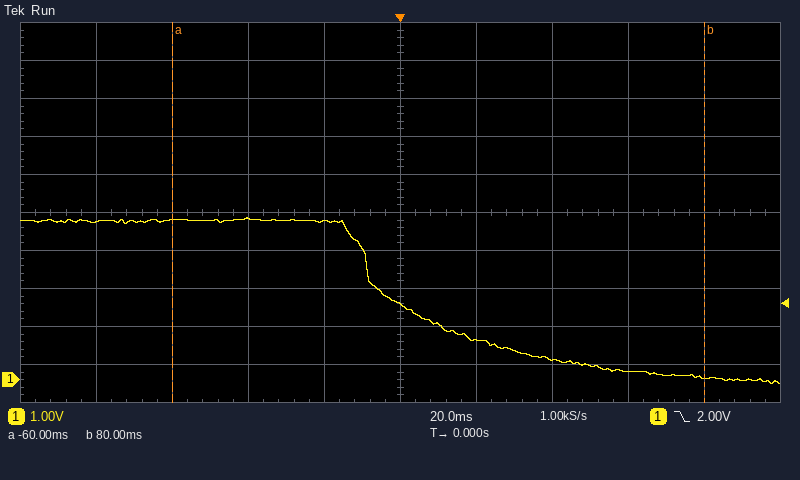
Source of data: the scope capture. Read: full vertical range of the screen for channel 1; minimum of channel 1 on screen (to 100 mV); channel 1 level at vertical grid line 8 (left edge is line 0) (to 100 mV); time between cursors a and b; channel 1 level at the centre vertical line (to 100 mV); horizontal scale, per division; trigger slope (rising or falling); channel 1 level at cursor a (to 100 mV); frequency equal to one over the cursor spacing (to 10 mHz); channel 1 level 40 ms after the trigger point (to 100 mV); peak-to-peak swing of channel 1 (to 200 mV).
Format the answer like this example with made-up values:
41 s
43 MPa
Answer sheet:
10 V
-100 mV
200 mV
140 ms
2.0 V
20 ms
falling
4.2 V
7.14 Hz
500 mV
4.4 V
